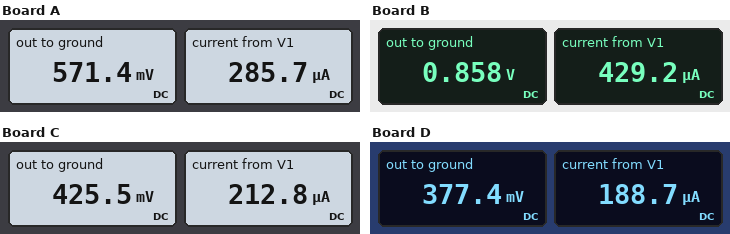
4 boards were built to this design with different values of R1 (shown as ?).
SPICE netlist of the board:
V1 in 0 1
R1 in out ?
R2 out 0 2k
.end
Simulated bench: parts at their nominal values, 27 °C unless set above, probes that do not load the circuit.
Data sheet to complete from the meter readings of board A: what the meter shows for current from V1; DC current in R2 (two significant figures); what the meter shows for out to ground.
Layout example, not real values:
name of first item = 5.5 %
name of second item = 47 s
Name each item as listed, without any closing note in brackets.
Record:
what the meter shows for current from V1 = 285.7 µA
DC current in R2 = 290 µA
what the meter shows for out to ground = 571.4 mV
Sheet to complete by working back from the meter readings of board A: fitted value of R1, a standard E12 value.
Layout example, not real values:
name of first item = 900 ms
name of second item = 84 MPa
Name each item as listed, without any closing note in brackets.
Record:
fitted value of R1, a standard E12 value = 1.5 kΩ
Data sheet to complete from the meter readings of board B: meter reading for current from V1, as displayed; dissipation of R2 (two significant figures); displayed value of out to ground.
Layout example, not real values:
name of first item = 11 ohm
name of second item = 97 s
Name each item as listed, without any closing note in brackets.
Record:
meter reading for current from V1, as displayed = 429.2 µA
dissipation of R2 = 370 µW
displayed value of out to ground = 0.858 V
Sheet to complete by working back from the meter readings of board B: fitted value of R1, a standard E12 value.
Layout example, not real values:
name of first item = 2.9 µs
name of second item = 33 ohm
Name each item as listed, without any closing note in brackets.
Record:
fitted value of R1, a standard E12 value = 330 Ω
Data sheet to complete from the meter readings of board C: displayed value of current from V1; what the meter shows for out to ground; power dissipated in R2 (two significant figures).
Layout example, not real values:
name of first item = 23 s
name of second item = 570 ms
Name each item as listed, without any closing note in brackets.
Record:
displayed value of current from V1 = 212.8 µA
what the meter shows for out to ground = 425.5 mV
power dissipated in R2 = 91 µW
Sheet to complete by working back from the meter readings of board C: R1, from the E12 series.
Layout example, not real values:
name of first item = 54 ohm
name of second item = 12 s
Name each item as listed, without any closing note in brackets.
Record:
R1, from the E12 series = 2.7 kΩ
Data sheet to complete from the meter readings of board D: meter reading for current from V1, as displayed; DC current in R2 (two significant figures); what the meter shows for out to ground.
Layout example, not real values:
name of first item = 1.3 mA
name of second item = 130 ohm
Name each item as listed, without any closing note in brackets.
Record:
meter reading for current from V1, as displayed = 188.7 µA
DC current in R2 = 190 µA
what the meter shows for out to ground = 377.4 mV
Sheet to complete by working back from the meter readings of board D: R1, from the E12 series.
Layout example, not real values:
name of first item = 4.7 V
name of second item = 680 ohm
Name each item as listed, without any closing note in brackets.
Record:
R1, from the E12 series = 3.3 kΩ
